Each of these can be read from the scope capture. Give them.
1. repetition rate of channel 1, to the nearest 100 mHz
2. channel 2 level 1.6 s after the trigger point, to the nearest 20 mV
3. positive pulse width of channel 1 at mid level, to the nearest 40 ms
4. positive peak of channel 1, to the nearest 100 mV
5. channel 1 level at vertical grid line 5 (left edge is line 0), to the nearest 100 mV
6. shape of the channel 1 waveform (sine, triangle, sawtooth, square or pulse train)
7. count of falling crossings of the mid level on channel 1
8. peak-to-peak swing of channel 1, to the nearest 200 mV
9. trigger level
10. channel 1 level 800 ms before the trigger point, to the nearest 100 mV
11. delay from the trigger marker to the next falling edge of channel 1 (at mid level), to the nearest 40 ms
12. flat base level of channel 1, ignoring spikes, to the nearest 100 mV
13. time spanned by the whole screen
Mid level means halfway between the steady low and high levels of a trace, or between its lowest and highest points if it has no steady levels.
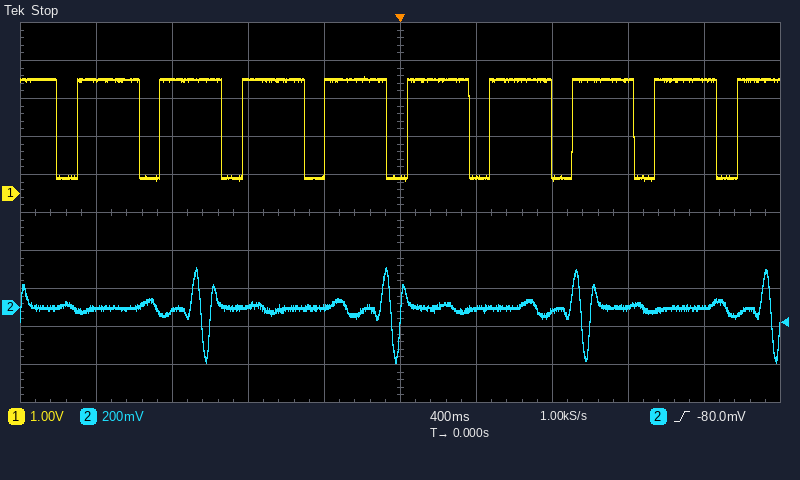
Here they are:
2.3 Hz
0 mV
320 ms
3.1 V
400 mV
pulse train
9
2.8 V
-80.0 mV
3.0 V
360 ms
400 mV
4 s
